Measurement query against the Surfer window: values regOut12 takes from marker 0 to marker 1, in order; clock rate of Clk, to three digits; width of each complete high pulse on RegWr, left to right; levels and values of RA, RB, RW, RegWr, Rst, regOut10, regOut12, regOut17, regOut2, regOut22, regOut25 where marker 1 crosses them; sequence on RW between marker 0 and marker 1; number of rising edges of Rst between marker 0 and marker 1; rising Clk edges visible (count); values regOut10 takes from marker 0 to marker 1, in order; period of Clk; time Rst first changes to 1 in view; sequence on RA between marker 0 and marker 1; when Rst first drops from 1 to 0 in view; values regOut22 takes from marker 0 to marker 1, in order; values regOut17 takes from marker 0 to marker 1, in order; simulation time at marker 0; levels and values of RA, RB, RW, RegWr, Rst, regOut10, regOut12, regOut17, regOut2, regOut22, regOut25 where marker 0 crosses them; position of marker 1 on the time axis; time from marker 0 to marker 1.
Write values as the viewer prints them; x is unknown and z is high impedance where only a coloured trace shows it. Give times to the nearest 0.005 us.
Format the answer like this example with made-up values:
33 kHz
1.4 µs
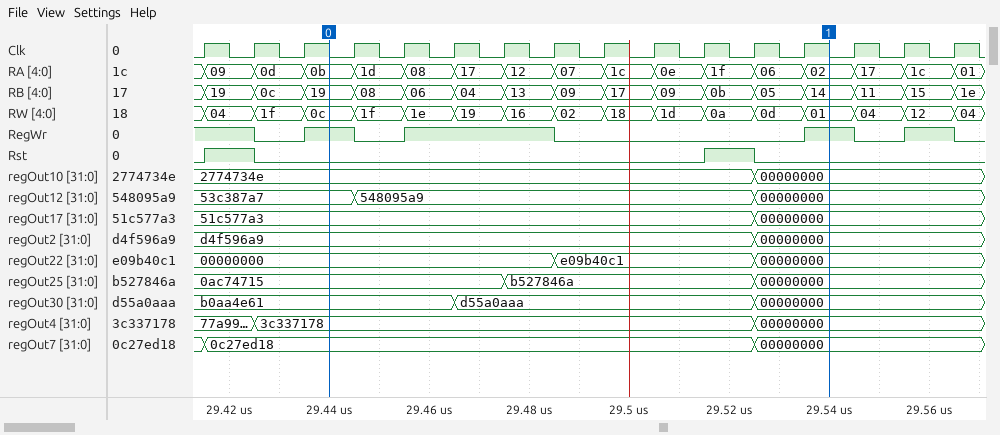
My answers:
53c387a7, 548095a9, 00000000
100 MHz
0.01 us, 0.03 us, 0.01 us, 0.01 us
RA=02, RB=14, RW=01, RegWr=1, Rst=0, regOut10=00000000, regOut12=00000000, regOut17=00000000, regOut2=00000000, regOut22=00000000, regOut25=00000000
0c, 1f, 1e, 19, 16, 02, 18, 1d, 0a, 0d, 01
1
16
2774734e, 00000000
0.01 us
29.415 us
0b, 1d, 08, 17, 12, 07, 1c, 0e, 1f, 06, 02
29.425 us
00000000, e09b40c1, 00000000
51c577a3, 00000000
29.44 us
RA=0b, RB=19, RW=0c, RegWr=1, Rst=0, regOut10=2774734e, regOut12=53c387a7, regOut17=51c577a3, regOut2=d4f596a9, regOut22=00000000, regOut25=0ac74715
29.54 us
0.1 us
